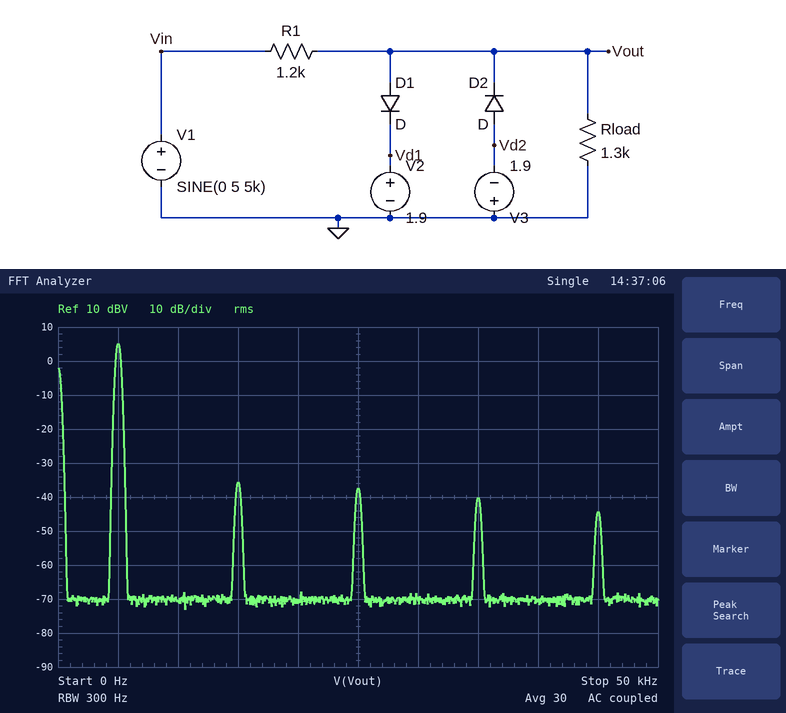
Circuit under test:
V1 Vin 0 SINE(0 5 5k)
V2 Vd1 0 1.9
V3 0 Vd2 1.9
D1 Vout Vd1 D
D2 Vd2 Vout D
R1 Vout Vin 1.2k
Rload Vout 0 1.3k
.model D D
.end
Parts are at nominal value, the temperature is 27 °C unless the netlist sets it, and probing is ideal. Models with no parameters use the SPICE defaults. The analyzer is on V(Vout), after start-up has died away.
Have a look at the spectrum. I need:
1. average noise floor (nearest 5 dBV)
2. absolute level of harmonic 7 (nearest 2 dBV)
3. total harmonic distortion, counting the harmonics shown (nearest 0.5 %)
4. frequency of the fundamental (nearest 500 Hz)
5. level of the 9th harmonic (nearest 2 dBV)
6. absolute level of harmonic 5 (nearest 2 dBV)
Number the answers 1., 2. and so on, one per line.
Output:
1. -70 dBV
2. -40 dBV
3. 1.5 %
4. 5.0 kHz
5. -44 dBV
6. -38 dBV
